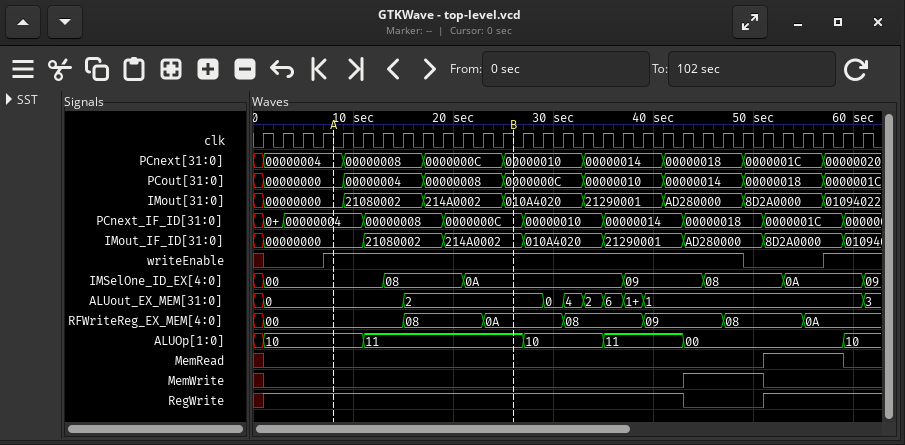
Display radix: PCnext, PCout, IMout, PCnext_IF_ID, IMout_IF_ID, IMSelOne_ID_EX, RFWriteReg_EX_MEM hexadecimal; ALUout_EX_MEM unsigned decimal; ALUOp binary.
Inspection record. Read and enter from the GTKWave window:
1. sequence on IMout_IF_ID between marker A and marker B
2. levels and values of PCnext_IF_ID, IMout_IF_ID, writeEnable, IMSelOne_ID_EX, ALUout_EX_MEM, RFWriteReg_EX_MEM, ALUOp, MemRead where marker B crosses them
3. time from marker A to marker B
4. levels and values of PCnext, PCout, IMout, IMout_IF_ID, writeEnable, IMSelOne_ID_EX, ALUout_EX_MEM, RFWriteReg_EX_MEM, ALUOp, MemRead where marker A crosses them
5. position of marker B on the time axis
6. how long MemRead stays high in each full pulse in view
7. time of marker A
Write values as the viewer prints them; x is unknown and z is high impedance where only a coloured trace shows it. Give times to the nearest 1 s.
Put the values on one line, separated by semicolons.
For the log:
00000000, 21080002, 214A0002; PCnext_IF_ID=0000000C, IMout_IF_ID=214A0002, writeEnable=1, IMSelOne_ID_EX=0A, ALUout_EX_MEM=2, RFWriteReg_EX_MEM=0A, ALUOp=11, MemRead=0; 18 s; PCnext=00000004, PCout=00000000, IMout=00000000, IMout_IF_ID=00000000, writeEnable=1, IMSelOne_ID_EX=00, ALUout_EX_MEM=0, RFWriteReg_EX_MEM=00, ALUOp=10, MemRead=0; 26 s; 8 s; 8 s
